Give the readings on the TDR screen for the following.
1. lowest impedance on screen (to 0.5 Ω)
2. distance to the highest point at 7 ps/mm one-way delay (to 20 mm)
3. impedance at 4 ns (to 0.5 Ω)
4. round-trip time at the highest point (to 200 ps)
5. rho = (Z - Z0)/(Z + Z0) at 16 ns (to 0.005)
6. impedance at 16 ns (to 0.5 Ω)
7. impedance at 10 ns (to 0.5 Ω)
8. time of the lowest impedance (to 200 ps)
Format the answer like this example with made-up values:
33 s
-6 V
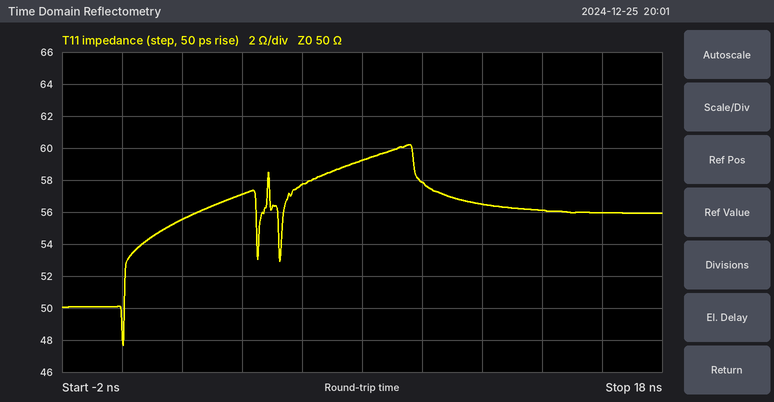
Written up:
47.5 Ω
680 mm
57.0 Ω
9.6 ns
+0.055
56.0 Ω
58.0 Ω
0.0 ns
